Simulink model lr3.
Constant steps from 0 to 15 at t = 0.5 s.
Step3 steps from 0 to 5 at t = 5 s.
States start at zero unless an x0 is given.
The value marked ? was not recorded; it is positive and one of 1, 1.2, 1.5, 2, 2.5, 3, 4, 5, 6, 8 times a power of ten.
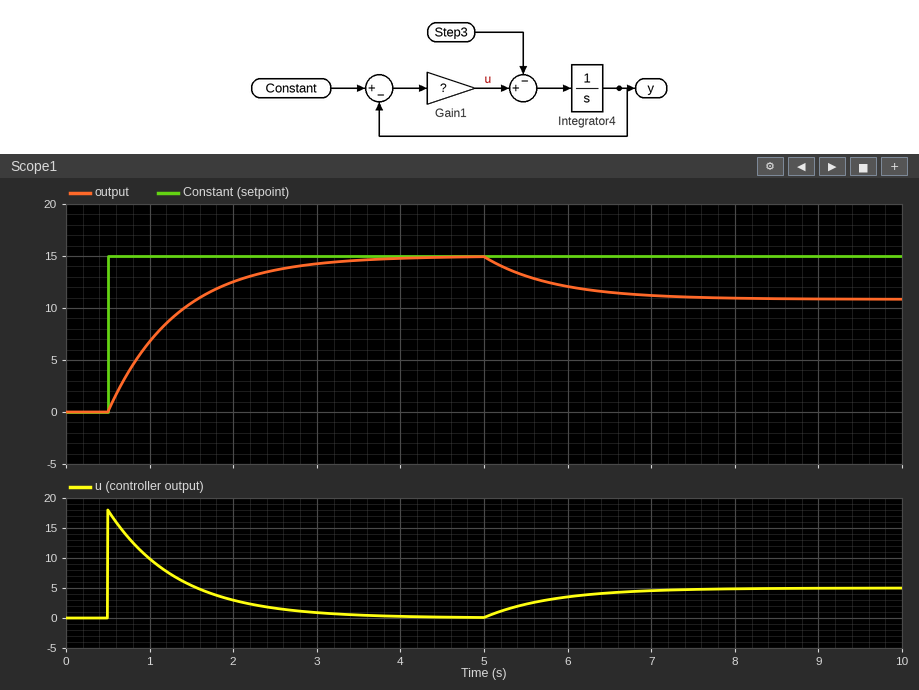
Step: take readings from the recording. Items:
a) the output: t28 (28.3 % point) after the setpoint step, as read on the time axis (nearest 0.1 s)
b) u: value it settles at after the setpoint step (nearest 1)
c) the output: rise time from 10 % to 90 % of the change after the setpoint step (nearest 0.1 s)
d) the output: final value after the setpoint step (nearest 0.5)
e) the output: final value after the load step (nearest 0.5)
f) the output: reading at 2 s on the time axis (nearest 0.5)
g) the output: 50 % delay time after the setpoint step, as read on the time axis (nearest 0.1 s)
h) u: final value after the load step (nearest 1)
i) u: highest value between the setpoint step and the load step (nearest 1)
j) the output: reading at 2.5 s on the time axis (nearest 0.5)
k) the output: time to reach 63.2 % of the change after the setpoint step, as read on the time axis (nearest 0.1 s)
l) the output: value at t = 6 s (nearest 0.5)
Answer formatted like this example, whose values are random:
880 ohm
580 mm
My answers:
0.8 s
0
1.8 s
15.0
11.0
12.5
1.1 s
5
18
13.5
1.3 s
12.0
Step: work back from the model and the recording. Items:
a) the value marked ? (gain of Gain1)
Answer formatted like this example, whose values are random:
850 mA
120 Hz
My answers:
1.2
